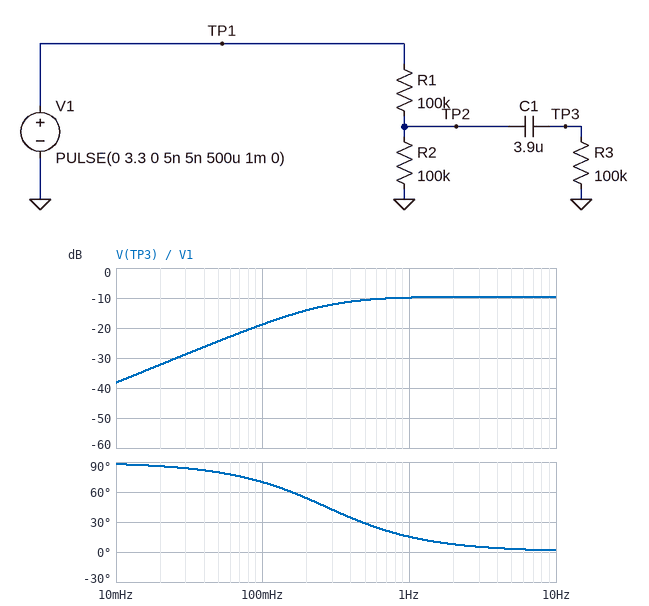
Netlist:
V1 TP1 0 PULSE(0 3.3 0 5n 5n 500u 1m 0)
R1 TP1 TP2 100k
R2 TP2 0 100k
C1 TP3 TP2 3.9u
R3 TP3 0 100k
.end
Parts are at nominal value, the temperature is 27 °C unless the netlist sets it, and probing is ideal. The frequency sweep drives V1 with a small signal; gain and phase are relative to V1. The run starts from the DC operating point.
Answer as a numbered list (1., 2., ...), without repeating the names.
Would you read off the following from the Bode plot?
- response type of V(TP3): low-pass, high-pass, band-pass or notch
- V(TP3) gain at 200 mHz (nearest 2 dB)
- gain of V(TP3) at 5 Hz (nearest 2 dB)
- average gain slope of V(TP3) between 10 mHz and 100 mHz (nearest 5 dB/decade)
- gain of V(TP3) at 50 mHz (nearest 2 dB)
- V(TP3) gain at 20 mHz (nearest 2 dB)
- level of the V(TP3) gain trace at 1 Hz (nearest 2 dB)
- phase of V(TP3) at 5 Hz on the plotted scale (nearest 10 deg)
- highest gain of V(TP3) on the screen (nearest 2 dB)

1. high-pass
2. -14 dB
3. -10 dB
4. 20 dB/decade
5. -24 dB
6. -32 dB
7. -10 dB
8. 0 deg
9. -10 dB
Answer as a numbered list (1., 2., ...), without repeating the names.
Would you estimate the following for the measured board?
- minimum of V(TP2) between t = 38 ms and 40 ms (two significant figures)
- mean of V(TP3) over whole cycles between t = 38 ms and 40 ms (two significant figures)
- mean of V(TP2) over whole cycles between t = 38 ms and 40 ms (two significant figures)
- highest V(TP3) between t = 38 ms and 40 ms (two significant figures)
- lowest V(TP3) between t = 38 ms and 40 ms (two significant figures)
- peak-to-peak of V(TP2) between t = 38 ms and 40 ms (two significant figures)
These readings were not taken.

1. 17 mV
2. 510 mV
3. 570 mV
4. 1.1 V
5. -36 mV
6. 1.1 V
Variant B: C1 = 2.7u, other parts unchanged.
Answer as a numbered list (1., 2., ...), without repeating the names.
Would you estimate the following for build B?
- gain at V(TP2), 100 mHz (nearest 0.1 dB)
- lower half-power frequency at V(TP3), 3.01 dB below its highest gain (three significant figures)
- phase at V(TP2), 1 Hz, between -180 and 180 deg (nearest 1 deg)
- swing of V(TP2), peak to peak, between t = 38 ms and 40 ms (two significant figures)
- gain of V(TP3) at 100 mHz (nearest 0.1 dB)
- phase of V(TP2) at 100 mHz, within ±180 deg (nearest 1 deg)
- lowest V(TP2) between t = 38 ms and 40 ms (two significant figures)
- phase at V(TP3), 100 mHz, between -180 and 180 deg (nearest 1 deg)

1. -6.2 dB
2. 393 mHz
3. -9 deg
4. 1.1 V
5. -21.7 dB
6. -5 deg
7. 25 mV
8. 76 deg
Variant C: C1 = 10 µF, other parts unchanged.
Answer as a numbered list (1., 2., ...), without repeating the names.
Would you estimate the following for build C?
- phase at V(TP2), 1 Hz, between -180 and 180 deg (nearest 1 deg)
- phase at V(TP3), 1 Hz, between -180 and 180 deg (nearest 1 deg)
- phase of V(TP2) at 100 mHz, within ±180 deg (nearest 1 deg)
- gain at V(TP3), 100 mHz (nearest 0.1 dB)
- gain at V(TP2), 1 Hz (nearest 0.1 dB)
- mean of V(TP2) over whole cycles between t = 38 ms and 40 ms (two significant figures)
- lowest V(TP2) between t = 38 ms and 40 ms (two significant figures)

1. -3 deg
2. 6 deg
3. -11 deg
4. -12.8 dB
5. -9.5 dB
6. 560 mV
7. 6.9 mV
